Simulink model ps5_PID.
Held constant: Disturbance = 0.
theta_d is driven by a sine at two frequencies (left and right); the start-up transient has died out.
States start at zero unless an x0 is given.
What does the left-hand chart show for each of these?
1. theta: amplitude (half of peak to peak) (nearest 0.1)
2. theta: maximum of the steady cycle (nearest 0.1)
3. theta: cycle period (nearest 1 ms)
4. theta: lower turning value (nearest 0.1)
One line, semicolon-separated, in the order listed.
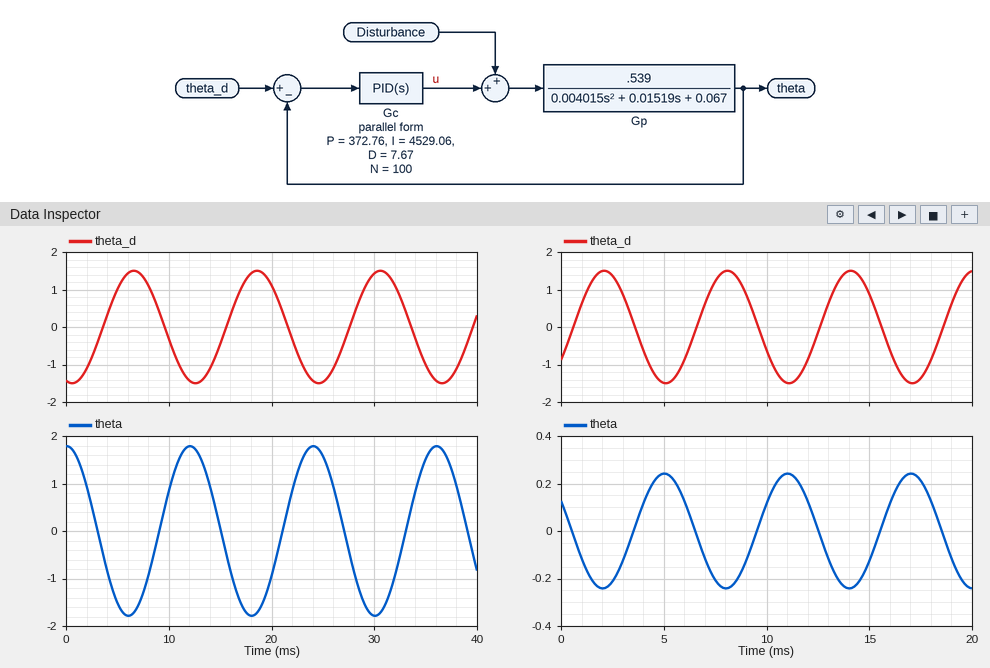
1.8; 1.8; 12 ms; -1.8
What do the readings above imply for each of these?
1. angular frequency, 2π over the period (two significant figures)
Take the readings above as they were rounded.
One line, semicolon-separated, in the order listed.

0.52 rad/ms
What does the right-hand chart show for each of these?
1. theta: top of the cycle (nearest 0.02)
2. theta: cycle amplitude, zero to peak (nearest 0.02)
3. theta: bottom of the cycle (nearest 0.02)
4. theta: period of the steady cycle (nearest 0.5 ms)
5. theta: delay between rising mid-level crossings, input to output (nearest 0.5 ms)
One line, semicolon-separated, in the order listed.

0.24; 0.24; -0.24; 6.0 ms; 3.0 ms
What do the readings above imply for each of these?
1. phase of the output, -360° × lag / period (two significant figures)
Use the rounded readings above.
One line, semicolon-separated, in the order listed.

-180°
